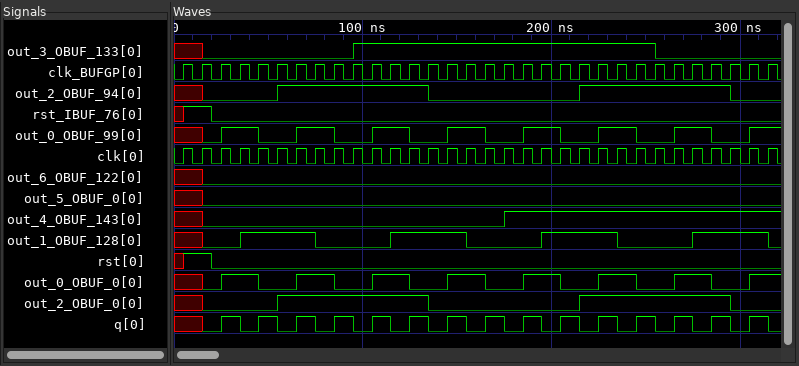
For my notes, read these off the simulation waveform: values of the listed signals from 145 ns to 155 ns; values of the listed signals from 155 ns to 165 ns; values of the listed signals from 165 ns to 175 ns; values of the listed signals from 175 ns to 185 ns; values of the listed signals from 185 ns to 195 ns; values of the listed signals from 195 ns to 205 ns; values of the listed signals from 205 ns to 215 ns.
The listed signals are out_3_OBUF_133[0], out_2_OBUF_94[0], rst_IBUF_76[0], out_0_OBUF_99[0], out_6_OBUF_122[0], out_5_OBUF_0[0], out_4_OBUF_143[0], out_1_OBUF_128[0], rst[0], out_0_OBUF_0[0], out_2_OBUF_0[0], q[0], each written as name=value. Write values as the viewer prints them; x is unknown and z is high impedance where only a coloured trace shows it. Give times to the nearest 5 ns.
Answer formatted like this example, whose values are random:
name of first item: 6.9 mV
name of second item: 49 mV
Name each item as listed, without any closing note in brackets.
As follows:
values of the listed signals from 145 ns to 155 ns: out_3_OBUF_133[0]=1, out_2_OBUF_94[0]=0, rst_IBUF_76[0]=0, out_0_OBUF_99[0]=1, out_6_OBUF_122[0]=0, out_5_OBUF_0[0]=0, out_4_OBUF_143[0]=0, out_1_OBUF_128[0]=1, rst[0]=0, out_0_OBUF_0[0]=1, out_2_OBUF_0[0]=0, q[0]=1
values of the listed signals from 155 ns to 165 ns: out_3_OBUF_133[0]=1, out_2_OBUF_94[0]=0, rst_IBUF_76[0]=0, out_0_OBUF_99[0]=1, out_6_OBUF_122[0]=0, out_5_OBUF_0[0]=0, out_4_OBUF_143[0]=0, out_1_OBUF_128[0]=0, rst[0]=0, out_0_OBUF_0[0]=1, out_2_OBUF_0[0]=0, q[0]=0
values of the listed signals from 165 ns to 175 ns: out_3_OBUF_133[0]=1, out_2_OBUF_94[0]=0, rst_IBUF_76[0]=0, out_0_OBUF_99[0]=0, out_6_OBUF_122[0]=0, out_5_OBUF_0[0]=0, out_4_OBUF_143[0]=0, out_1_OBUF_128[0]=0, rst[0]=0, out_0_OBUF_0[0]=0, out_2_OBUF_0[0]=0, q[0]=1
values of the listed signals from 175 ns to 185 ns: out_3_OBUF_133[0]=1, out_2_OBUF_94[0]=0, rst_IBUF_76[0]=0, out_0_OBUF_99[0]=0, out_6_OBUF_122[0]=0, out_5_OBUF_0[0]=0, out_4_OBUF_143[0]=1, out_1_OBUF_128[0]=0, rst[0]=0, out_0_OBUF_0[0]=0, out_2_OBUF_0[0]=0, q[0]=0
values of the listed signals from 185 ns to 195 ns: out_3_OBUF_133[0]=1, out_2_OBUF_94[0]=0, rst_IBUF_76[0]=0, out_0_OBUF_99[0]=1, out_6_OBUF_122[0]=0, out_5_OBUF_0[0]=0, out_4_OBUF_143[0]=1, out_1_OBUF_128[0]=0, rst[0]=0, out_0_OBUF_0[0]=1, out_2_OBUF_0[0]=0, q[0]=1
values of the listed signals from 195 ns to 205 ns: out_3_OBUF_133[0]=1, out_2_OBUF_94[0]=0, rst_IBUF_76[0]=0, out_0_OBUF_99[0]=1, out_6_OBUF_122[0]=0, out_5_OBUF_0[0]=0, out_4_OBUF_143[0]=1, out_1_OBUF_128[0]=1, rst[0]=0, out_0_OBUF_0[0]=1, out_2_OBUF_0[0]=0, q[0]=0
values of the listed signals from 205 ns to 215 ns: out_3_OBUF_133[0]=1, out_2_OBUF_94[0]=0, rst_IBUF_76[0]=0, out_0_OBUF_99[0]=0, out_6_OBUF_122[0]=0, out_5_OBUF_0[0]=0, out_4_OBUF_143[0]=1, out_1_OBUF_128[0]=1, rst[0]=0, out_0_OBUF_0[0]=0, out_2_OBUF_0[0]=0, q[0]=1
